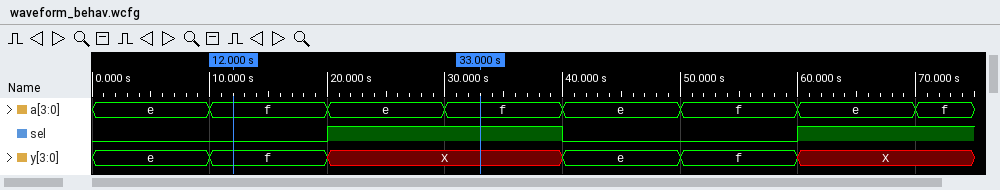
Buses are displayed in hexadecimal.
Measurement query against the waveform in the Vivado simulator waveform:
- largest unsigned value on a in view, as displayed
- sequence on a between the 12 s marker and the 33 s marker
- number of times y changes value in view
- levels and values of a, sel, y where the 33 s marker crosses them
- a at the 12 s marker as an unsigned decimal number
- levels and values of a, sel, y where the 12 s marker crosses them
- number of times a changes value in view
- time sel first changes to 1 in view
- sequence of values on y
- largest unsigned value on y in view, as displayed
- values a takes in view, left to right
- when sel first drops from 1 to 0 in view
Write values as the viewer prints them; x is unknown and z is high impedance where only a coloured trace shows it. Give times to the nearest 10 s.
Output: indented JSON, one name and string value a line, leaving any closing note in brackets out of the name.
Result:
{
  "largest unsigned value on a in view, as displayed": "f",
  "sequence on a between the 12 s marker and the 33 s marker": "f, e, f",
  "number of times y changes value in view": "5",
  "levels and values of a, sel, y where the 33 s marker crosses them": "a=f, sel=1, y=X",
  "a at the 12 s marker as an unsigned decimal number": "15",
  "levels and values of a, sel, y where the 12 s marker crosses them": "a=f, sel=0, y=f",
  "number of times a changes value in view": "7",
  "time sel first changes to 1 in view": "20 s",
  "sequence of values on y": "e, f, X, e, f, X",
  "largest unsigned value on y in view, as displayed": "f",
  "values a takes in view, left to right": "e, f, e, f, e, f, e, f",
  "when sel first drops from 1 to 0 in view": "40 s"
}
